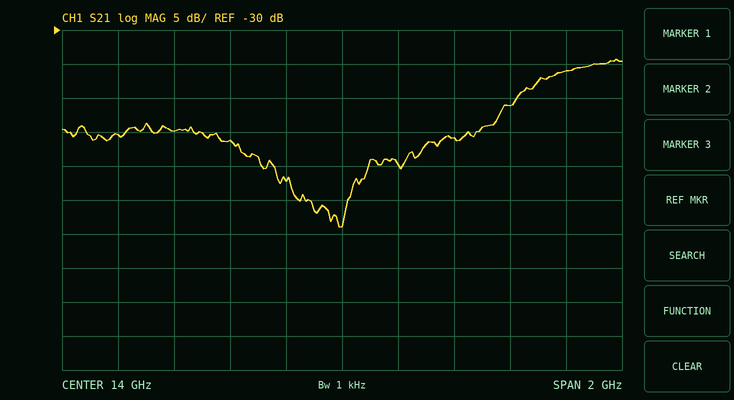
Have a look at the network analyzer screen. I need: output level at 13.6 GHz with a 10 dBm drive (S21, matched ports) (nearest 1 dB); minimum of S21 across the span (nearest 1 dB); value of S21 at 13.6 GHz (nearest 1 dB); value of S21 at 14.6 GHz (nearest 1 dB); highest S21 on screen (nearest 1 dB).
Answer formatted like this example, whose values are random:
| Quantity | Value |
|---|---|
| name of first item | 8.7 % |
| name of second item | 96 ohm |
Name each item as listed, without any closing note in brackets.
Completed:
| Quantity | Value |
|---|---|
| output level at 13.6 GHz with a 10 dBm drive (S21, matched ports) | -36 dBm |
| minimum of S21 across the span | -59 dB |
| value of S21 at 13.6 GHz | -46 dB |
| value of S21 at 14.6 GHz | -41 dB |
| highest S21 on screen | -34 dB |
